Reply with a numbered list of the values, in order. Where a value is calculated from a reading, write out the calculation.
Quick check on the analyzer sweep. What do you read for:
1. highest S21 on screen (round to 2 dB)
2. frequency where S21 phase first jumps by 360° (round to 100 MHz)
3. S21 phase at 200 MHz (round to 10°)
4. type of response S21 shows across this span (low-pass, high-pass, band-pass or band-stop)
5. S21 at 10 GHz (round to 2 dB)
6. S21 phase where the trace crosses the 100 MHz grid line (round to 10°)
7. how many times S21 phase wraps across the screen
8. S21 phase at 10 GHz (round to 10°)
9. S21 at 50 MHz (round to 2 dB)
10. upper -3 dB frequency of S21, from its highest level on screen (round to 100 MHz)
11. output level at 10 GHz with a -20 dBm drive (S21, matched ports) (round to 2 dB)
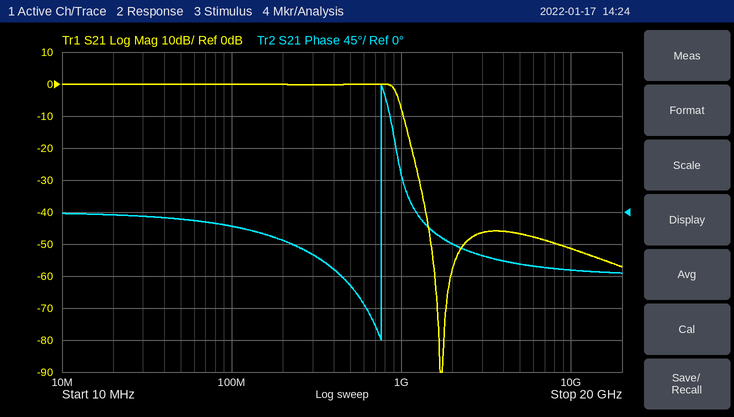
1. 0 dB
2. 800 MHz
3. -40°
4. low-pass
5. -52 dB
6. -20°
7. 1
8. -80°
9. 0 dB
10. 900 MHz
11. -20 dBm + (-52 dB) = -72 dBm
